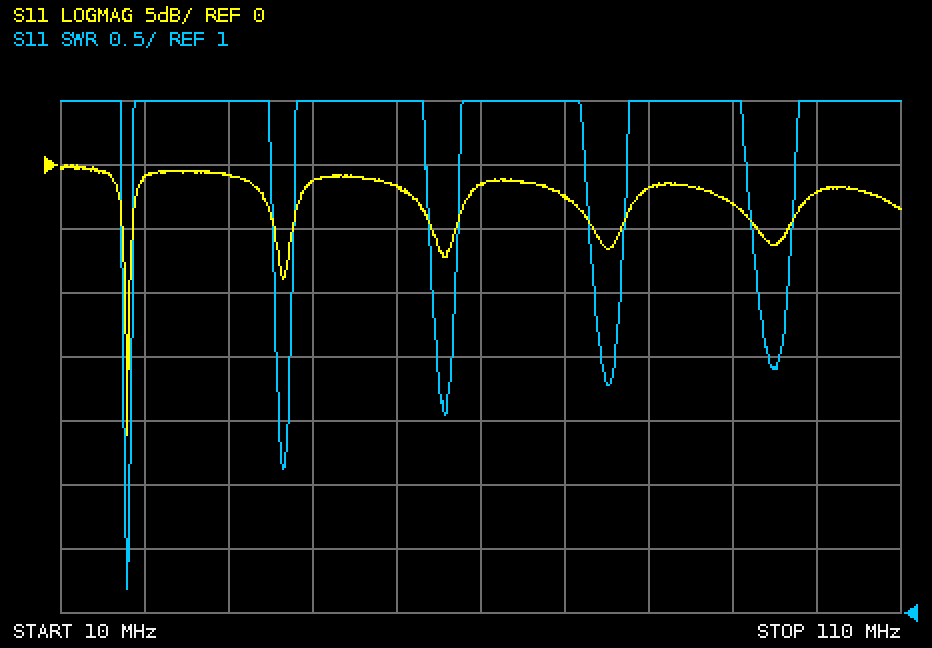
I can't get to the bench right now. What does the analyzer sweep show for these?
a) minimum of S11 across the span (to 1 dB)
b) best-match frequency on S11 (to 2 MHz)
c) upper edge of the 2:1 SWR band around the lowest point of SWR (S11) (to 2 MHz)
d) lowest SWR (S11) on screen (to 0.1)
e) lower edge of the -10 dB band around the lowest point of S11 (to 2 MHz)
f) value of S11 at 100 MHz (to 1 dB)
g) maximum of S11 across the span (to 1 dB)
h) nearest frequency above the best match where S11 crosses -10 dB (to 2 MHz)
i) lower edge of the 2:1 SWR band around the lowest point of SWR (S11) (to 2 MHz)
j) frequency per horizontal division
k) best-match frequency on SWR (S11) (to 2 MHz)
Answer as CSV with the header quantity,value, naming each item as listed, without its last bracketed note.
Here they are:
quantity,value
minimum of S11 across the span,-21 dB
best-match frequency on S11,18 MHz
upper edge of the 2:1 SWR band around the lowest point of SWR (S11),18 MHz
lowest SWR (S11) on screen,1.2
lower edge of the -10 dB band around the lowest point of S11,18 MHz
value of S11 at 100 MHz,-2 dB
maximum of S11 across the span,0 dB
nearest frequency above the best match where S11 crosses -10 dB,18 MHz
lower edge of the 2:1 SWR band around the lowest point of SWR (S11),18 MHz
frequency per horizontal division,10 MHz
best-match frequency on SWR (S11),18 MHz
